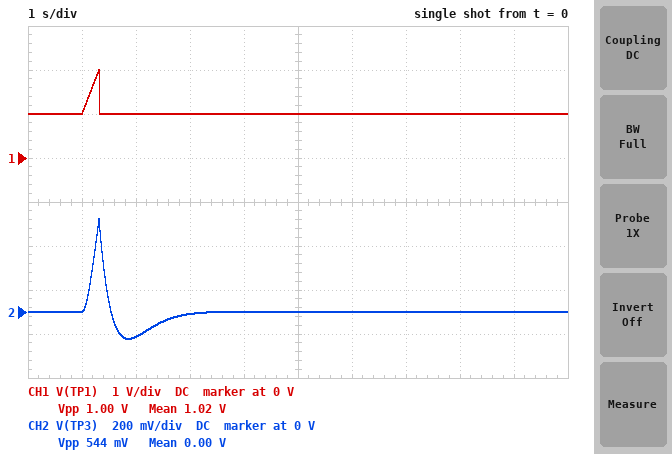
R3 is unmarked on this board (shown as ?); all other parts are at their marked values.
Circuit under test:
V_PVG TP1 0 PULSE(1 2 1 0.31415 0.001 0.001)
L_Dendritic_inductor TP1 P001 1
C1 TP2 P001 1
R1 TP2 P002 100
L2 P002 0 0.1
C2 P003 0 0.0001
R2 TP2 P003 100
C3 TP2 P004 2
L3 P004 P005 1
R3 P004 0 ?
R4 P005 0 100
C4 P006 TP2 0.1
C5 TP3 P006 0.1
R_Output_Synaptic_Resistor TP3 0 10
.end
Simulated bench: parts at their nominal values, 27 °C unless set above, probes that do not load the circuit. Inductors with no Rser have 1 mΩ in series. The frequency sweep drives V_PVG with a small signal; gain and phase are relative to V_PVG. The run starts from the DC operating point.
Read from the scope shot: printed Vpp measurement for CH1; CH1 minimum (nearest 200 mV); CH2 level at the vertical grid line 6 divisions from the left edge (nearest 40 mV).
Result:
1.00 V
1.0 V
0 V
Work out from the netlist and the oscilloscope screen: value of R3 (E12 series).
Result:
12 Ω
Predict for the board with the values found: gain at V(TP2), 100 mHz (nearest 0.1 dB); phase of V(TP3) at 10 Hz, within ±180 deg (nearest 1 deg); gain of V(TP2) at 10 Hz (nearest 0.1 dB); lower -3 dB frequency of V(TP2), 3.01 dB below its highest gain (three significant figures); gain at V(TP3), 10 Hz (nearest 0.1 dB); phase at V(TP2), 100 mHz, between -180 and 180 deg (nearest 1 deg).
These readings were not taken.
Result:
-0.3 dB
-84 deg
-22.1 dB
25.2 mHz
-22.1 dB
6 deg
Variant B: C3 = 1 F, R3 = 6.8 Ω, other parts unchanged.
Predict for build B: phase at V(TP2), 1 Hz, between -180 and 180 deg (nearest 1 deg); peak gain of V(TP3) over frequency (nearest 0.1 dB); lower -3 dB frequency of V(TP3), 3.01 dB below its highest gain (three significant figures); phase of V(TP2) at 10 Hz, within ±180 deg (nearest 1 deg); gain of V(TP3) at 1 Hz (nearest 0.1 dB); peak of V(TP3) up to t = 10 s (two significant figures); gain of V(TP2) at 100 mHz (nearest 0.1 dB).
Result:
-63 deg
-2.1 dB
205 mHz
-87 deg
-5.4 dB
350 mV
-0.6 dB
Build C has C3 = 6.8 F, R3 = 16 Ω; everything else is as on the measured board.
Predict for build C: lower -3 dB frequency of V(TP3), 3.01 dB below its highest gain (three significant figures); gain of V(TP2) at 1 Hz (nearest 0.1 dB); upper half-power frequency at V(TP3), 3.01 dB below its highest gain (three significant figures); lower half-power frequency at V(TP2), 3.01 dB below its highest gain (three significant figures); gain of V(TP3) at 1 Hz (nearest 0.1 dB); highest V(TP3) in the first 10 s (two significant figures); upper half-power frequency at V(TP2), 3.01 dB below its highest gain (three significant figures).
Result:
235 mHz
-2.6 dB
1.24 Hz
17.5 mHz
-3.0 dB
450 mV
991 mHz
